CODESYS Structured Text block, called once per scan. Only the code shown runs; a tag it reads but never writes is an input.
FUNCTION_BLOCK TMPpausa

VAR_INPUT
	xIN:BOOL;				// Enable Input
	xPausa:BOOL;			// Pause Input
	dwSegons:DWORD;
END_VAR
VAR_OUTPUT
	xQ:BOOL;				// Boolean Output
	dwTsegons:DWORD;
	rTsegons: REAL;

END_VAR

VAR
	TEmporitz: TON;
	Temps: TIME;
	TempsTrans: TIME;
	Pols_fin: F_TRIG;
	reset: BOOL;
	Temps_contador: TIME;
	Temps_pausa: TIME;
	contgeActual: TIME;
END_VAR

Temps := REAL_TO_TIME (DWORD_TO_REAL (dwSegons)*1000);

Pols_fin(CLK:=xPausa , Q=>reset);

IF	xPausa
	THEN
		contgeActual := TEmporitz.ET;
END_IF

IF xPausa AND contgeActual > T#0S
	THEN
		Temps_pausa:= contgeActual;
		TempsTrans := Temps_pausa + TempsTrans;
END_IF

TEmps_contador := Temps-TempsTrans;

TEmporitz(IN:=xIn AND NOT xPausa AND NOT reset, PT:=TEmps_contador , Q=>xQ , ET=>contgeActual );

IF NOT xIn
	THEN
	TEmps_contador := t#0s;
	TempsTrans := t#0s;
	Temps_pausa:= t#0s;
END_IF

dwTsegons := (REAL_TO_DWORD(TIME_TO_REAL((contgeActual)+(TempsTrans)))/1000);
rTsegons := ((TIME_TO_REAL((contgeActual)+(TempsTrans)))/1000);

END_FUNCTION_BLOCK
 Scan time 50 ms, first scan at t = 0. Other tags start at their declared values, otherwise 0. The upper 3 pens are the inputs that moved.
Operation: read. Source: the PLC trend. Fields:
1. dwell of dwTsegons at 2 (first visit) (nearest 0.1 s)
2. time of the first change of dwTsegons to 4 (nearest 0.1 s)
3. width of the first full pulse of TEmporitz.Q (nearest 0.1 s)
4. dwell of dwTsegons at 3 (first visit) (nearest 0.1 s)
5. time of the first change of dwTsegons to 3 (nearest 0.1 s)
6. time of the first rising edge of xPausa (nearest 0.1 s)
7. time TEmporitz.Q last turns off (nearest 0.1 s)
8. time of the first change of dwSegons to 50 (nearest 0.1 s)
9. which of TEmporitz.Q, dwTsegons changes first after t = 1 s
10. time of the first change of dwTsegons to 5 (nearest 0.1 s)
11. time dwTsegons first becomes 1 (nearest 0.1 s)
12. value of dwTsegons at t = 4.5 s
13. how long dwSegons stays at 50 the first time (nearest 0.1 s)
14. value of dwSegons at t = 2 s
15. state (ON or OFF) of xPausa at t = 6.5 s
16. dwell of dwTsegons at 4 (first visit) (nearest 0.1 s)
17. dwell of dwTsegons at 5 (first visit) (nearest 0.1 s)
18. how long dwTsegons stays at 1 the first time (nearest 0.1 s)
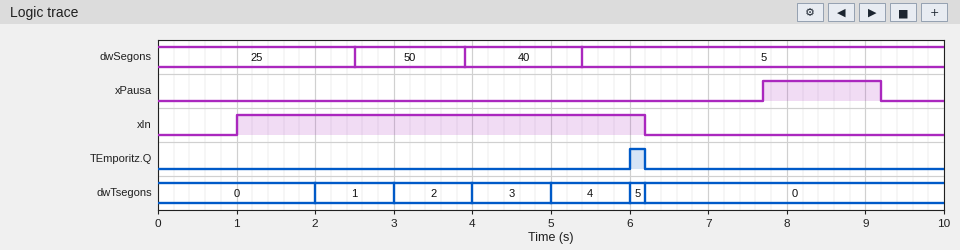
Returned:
1.0 s
5.0 s
0.2 s
1.0 s
4.0 s
7.7 s
6.2 s
2.5 s
dwTsegons
6.0 s
2.0 s
3
1.4 s
25
OFF
1.0 s
0.2 s
1.0 s
